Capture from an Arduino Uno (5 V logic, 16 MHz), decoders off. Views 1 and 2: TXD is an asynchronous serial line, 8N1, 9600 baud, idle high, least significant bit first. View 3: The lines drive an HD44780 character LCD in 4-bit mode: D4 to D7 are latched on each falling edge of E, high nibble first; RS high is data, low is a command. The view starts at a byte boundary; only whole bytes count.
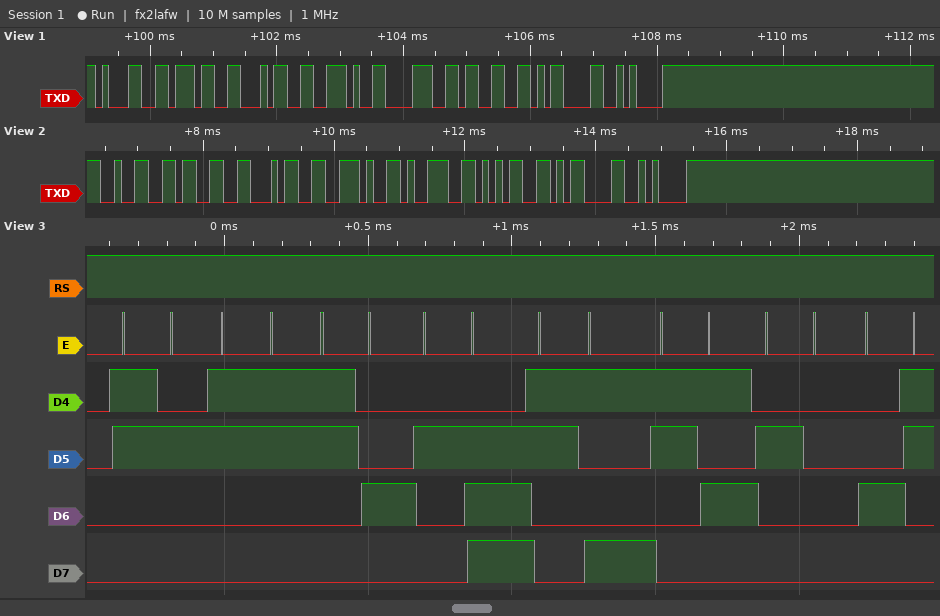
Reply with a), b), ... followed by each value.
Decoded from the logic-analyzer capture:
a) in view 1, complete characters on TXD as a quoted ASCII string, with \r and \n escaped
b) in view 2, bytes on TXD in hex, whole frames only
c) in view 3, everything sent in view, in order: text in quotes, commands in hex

a) "174.83\r\n"
b) 0x32 0x33 0x34 0x2E 0x39 0x35 0x0D 0x0A
c) "234.95 C"
